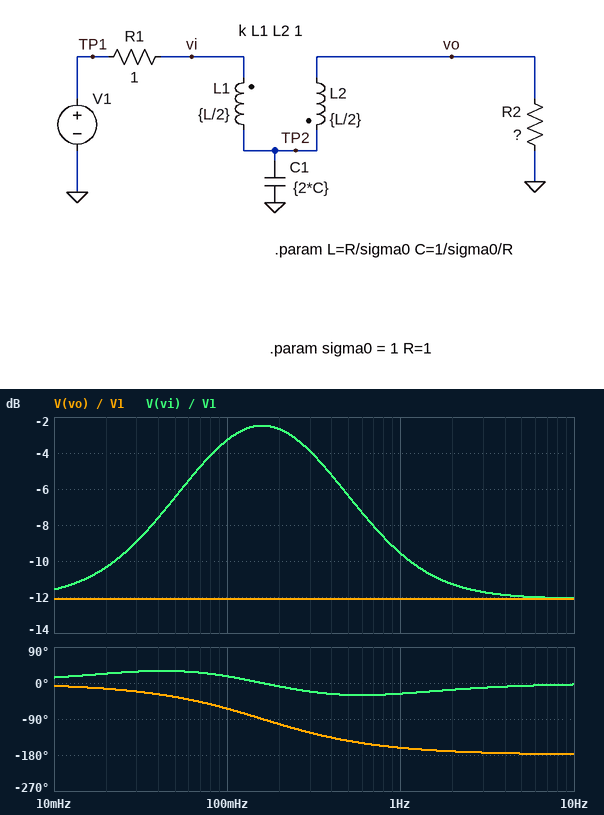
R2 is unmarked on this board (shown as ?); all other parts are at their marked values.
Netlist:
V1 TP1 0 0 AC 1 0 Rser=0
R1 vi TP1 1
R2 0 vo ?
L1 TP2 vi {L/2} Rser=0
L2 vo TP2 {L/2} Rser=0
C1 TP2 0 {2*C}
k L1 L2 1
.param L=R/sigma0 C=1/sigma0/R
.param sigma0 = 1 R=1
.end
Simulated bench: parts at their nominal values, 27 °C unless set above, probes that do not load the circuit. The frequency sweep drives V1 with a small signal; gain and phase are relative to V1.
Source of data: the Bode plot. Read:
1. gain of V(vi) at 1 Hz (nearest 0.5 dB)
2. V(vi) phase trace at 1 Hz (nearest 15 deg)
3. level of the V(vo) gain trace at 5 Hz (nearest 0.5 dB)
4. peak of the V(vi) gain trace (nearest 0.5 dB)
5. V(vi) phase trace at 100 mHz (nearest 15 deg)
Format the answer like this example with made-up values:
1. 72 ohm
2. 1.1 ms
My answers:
1. -9.5 dB
2. -30 deg
3. -12.0 dB
4. -2.5 dB
5. 15 deg
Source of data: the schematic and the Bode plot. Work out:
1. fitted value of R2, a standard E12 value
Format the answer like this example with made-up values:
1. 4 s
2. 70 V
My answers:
1. 0.33 Ω
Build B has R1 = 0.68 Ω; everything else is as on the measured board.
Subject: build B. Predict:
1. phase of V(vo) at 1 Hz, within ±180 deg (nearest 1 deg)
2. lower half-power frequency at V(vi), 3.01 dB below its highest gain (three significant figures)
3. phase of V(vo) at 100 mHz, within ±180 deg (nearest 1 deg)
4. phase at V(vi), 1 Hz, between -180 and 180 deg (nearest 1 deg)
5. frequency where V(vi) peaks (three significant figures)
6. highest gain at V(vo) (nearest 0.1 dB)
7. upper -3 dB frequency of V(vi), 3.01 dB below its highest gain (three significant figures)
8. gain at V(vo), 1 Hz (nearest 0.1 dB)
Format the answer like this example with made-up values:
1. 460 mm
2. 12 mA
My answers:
1. -158 deg
2. 49.0 mHz
3. -68 deg
4. -23 deg
5. 159 mHz
6. -9.7 dB
7. 517 mHz
8. -9.9 dB
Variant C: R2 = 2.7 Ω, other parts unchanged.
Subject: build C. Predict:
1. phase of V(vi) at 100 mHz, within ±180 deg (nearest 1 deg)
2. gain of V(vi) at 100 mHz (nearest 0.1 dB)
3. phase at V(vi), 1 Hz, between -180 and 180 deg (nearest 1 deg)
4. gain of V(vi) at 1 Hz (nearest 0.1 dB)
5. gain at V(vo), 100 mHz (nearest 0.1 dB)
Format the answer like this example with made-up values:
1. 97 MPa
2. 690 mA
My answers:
1. -27 deg
2. -8.0 dB
3. 11 deg
4. -3.1 dB
5. -2.7 dB
